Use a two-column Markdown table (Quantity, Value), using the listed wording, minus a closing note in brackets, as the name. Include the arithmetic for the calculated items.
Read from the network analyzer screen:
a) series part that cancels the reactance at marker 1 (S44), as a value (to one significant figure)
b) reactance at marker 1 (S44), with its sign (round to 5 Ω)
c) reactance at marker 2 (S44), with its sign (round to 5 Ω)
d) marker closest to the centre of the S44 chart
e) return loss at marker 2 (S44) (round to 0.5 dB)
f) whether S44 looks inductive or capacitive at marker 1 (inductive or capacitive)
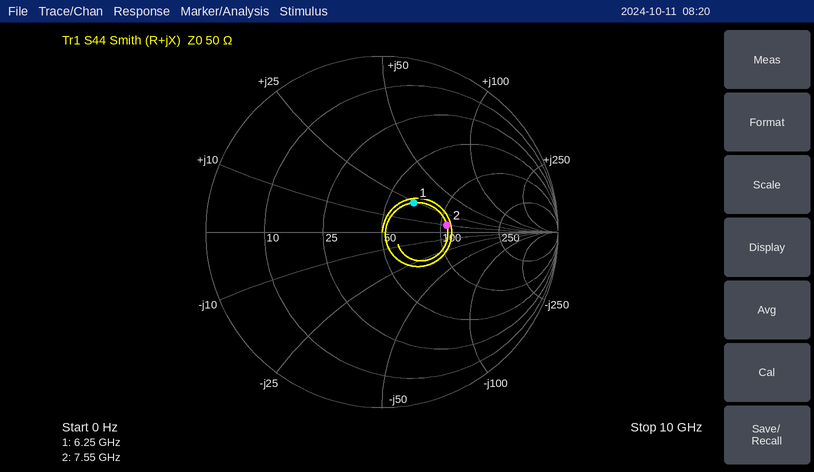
| Quantity | Value |
|---|---|
| series part that cancels the reactance at marker 1 (S44), as a value | C = 1/(2π × 6.25 GHz × 25 Ω) ≈ 1 pF |
| reactance at marker 1 (S44), with its sign | +25 Ω |
| reactance at marker 2 (S44), with its sign | +10 Ω |
| marker closest to the centre of the S44 chart | marker 1 |
| return loss at marker 2 (S44) | 8.5 dB |
| whether S44 looks inductive or capacitive at marker 1 | inductive |
